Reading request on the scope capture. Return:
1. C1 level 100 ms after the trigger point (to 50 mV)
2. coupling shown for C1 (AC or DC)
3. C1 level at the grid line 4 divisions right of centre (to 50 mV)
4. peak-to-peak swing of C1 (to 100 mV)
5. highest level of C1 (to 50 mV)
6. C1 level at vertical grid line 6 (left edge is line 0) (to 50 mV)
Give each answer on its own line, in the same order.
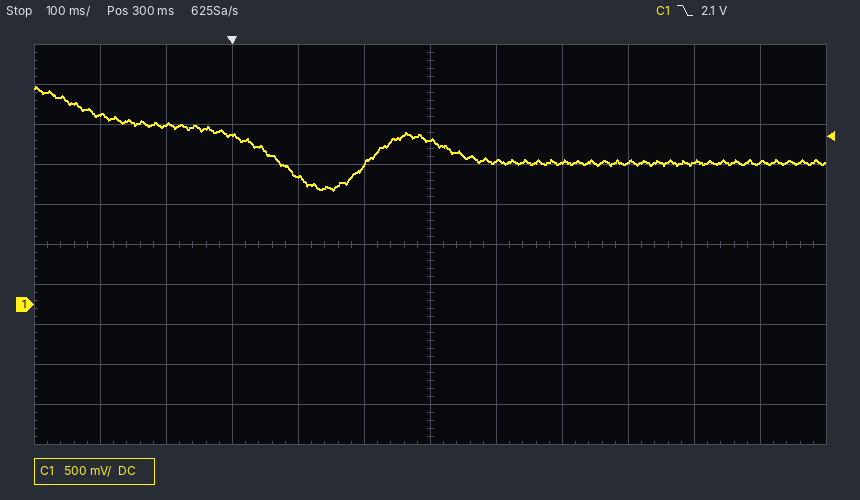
1.60 V
DC
1.80 V
1.30 V
2.70 V
2.05 V
